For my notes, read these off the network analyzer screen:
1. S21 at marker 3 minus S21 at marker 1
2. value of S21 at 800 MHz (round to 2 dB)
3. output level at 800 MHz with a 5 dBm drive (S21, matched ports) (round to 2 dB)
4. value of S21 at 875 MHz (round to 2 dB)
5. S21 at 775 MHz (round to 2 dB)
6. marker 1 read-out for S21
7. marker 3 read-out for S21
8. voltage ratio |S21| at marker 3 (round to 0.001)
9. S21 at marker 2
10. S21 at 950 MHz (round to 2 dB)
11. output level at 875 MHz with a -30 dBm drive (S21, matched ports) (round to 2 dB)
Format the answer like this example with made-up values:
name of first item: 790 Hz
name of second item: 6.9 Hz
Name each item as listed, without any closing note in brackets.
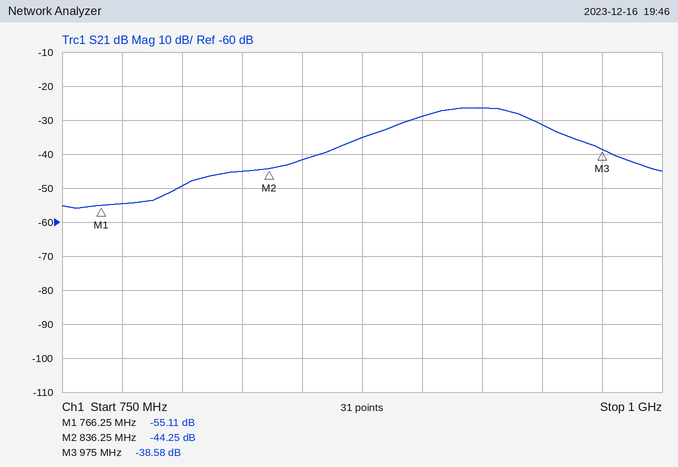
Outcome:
S21 at marker 3 minus S21 at marker 1: 16.53 dB
value of S21 at 800 MHz: -50 dB
output level at 800 MHz with a 5 dBm drive (S21, matched ports): -44 dBm
value of S21 at 875 MHz: -36 dB
S21 at 775 MHz: -54 dB
marker 1 read-out for S21: -55.11 dB
marker 3 read-out for S21: -38.58 dB
voltage ratio |S21| at marker 3: 0.012
S21 at marker 2: -44.25 dB
S21 at 950 MHz: -32 dB
output level at 875 MHz with a -30 dBm drive (S21, matched ports): -66 dBm
